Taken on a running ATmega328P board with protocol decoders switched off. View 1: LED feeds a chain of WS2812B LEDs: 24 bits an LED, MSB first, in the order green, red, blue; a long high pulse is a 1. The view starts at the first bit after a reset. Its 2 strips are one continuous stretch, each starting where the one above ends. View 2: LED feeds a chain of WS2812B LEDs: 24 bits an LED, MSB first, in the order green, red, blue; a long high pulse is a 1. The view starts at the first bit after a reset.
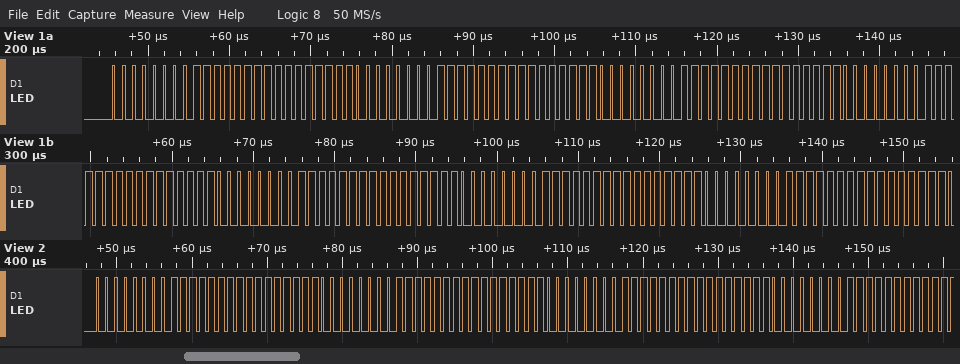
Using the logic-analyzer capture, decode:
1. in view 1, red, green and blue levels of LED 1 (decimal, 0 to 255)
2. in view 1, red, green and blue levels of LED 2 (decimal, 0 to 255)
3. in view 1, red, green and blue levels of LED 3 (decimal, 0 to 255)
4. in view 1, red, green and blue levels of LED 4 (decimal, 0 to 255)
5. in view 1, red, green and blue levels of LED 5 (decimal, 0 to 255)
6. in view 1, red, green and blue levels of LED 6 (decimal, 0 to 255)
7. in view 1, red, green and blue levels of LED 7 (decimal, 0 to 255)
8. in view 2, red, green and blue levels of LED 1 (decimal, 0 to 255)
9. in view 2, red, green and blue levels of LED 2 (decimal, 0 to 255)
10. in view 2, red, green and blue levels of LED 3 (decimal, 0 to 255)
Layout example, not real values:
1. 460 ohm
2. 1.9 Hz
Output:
1. 255, 0, 255
2. 255, 0, 255
3. 255, 0, 255
4. 255, 0, 255
5. 255, 0, 255
6. 255, 0, 255
7. 255, 0, 255
8. 255, 0, 255
9. 255, 0, 255
10. 255, 0, 255
